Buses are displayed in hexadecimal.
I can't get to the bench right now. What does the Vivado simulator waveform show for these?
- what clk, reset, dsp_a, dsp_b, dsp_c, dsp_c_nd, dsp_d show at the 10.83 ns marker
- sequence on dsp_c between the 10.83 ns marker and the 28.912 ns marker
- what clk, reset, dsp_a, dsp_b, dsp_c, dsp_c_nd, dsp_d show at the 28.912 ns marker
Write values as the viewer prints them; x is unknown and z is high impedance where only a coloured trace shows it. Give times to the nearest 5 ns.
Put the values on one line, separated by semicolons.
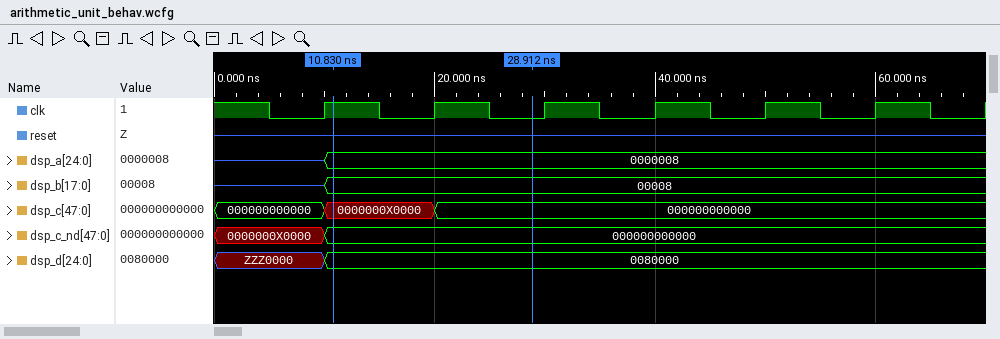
clk=1, reset=z, dsp_a=0000008, dsp_b=00008, dsp_c=0000000X0000, dsp_c_nd=000000000000, dsp_d=0080000; 0000000X0000, 000000000000; clk=0, reset=z, dsp_a=0000008, dsp_b=00008, dsp_c=000000000000, dsp_c_nd=000000000000, dsp_d=0080000
